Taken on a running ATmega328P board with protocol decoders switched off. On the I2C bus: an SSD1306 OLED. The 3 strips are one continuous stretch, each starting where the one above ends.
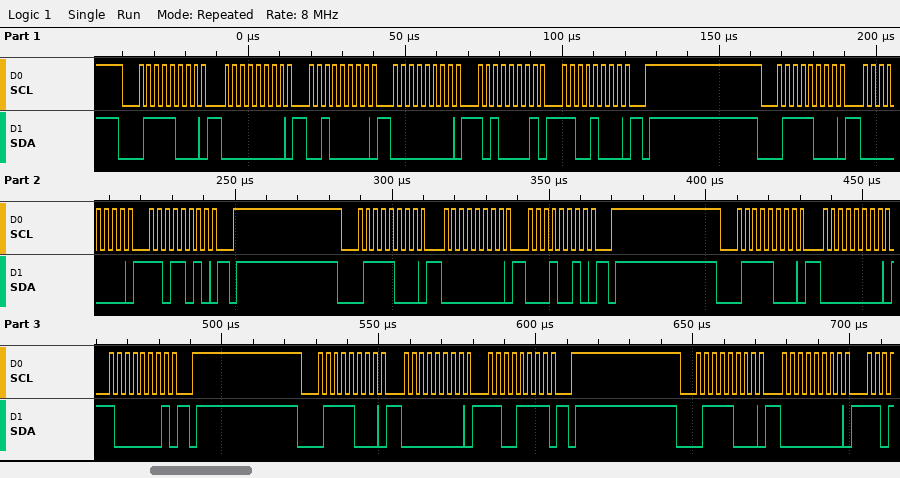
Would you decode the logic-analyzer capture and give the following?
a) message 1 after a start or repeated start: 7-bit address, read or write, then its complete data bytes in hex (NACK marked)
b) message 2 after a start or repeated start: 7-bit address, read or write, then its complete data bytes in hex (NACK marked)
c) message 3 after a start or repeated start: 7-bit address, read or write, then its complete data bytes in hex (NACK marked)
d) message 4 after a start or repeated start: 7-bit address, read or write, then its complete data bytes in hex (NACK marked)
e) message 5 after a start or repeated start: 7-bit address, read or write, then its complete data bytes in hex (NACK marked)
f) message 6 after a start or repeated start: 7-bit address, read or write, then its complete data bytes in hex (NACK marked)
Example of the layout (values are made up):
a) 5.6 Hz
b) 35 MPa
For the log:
a) 0x3C write: 00 20 00 A1 C8
b) 0x3C write: 00 DA
c) 0x3C write: 00 12
d) 0x3C write: 00 81
e) 0x3C write: 00 CF
f) 0x3C write: 00
